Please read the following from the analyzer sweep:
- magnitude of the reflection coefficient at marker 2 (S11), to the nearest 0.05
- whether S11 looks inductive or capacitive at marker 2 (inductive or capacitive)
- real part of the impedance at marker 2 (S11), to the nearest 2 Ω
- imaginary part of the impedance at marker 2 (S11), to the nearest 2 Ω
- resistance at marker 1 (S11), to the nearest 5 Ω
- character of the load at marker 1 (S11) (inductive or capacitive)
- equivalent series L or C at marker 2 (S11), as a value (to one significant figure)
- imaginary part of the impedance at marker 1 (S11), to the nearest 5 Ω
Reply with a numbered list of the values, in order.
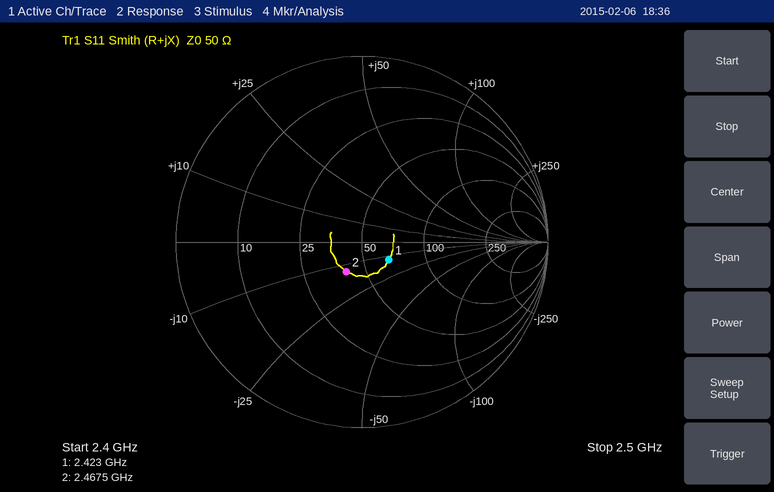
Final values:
1. 0.20
2. capacitive
3. 40 Ω
4. -14 Ω
5. 65 Ω
6. capacitive
7. 5 pF
8. -15 Ω
